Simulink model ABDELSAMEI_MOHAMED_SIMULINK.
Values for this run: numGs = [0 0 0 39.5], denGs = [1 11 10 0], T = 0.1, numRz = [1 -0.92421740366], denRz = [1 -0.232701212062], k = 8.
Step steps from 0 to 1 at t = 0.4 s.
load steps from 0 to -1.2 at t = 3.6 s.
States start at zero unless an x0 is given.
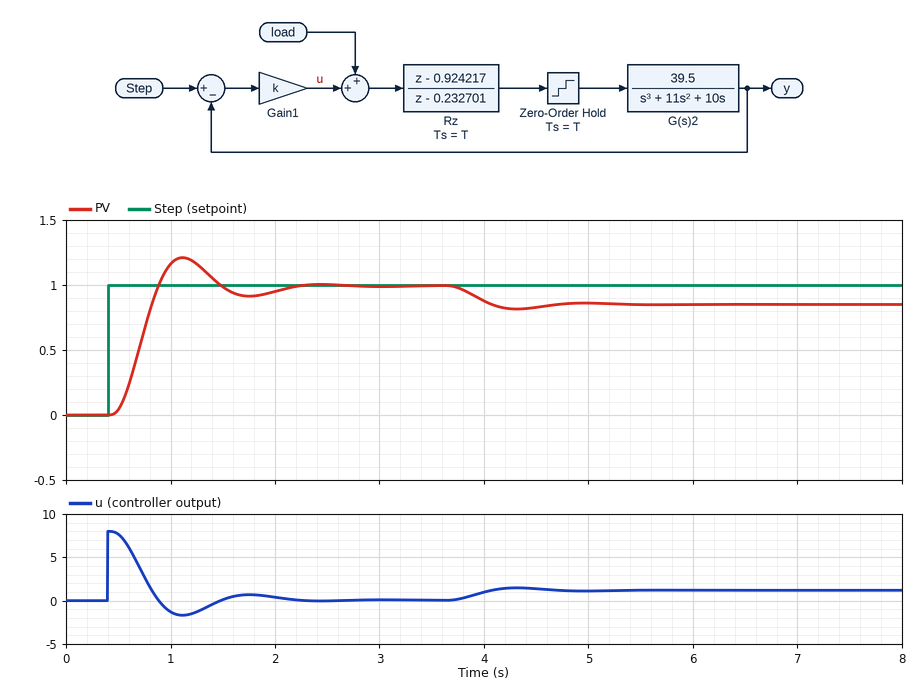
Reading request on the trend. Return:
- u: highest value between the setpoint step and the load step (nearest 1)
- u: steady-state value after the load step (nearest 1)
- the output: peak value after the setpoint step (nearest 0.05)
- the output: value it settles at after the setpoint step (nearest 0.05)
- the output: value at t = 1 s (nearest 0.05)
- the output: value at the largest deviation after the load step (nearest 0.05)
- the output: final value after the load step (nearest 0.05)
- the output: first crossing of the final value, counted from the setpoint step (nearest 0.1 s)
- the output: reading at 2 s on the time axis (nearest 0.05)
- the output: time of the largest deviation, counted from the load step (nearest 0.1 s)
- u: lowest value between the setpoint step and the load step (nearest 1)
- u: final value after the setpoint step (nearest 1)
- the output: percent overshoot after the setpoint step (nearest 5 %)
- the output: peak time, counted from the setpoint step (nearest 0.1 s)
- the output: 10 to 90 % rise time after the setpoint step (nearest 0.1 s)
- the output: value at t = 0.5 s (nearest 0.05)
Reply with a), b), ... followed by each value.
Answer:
a) 8
b) 1
c) 1.20
d) 1.00
e) 1.15
f) 0.80
g) 0.85
h) 0.5 s
i) 0.95
j) 0.7 s
k) -2
l) 0
m) 20 %
n) 0.7 s
o) 0.3 s
p) 0.05
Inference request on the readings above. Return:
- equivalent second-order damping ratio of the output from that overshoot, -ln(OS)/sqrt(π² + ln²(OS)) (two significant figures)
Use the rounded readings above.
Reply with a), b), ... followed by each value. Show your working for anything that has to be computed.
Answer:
a) ln(0.2) = -1.609; 1.609 / sqrt(9.870 + 2.590) = 0.46
